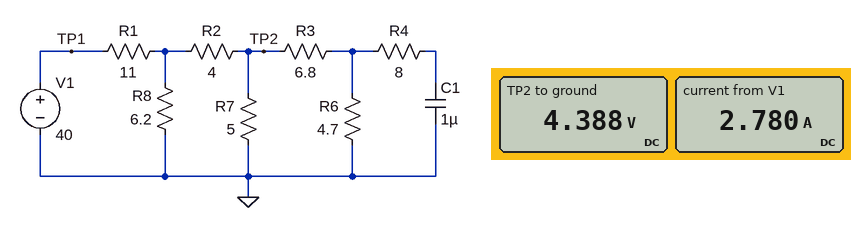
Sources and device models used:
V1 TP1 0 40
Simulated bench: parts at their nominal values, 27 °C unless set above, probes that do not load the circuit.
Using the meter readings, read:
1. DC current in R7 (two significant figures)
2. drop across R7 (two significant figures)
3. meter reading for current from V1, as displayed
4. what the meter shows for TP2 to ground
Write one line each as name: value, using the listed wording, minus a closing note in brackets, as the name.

DC current in R7: 880 mA
drop across R7: 4.4 V
meter reading for current from V1, as displayed: 2.780 A
what the meter shows for TP2 to ground: 4.388 V
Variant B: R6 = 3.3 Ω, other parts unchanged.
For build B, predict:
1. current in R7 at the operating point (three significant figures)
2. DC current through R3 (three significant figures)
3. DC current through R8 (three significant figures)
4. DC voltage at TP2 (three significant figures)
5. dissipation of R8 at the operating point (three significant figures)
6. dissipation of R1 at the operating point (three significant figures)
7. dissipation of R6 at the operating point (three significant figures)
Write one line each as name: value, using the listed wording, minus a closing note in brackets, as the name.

current in R7 at the operating point: 853 mA
DC current through R3: 422 mA
DC current through R8: 1.51 A
DC voltage at TP2: 4.26 V
dissipation of R8 at the operating point: 14.1 W
dissipation of R1 at the operating point: 85.3 W
dissipation of R6 at the operating point: 588 mW
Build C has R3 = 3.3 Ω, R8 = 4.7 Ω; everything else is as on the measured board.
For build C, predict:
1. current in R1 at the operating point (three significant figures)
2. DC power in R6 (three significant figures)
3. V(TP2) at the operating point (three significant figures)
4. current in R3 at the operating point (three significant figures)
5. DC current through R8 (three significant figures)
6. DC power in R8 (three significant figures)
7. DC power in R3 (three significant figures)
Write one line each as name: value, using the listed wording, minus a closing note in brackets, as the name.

current in R1 at the operating point: 2.89 A
DC power in R6: 927 mW
V(TP2) at the operating point: 3.55 V
current in R3 at the operating point: 444 mA
DC current through R8: 1.74 A
DC power in R8: 14.2 W
DC power in R3: 651 mW
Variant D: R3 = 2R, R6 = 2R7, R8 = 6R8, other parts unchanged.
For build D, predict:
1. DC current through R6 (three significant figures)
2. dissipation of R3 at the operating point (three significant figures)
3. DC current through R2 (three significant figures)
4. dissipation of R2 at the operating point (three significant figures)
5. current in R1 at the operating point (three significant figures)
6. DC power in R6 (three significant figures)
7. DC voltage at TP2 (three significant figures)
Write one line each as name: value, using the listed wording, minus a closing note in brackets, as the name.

DC current through R6: 741 mA
dissipation of R3 at the operating point: 1.10 W
DC current through R2: 1.44 A
dissipation of R2 at the operating point: 8.27 W
current in R1 at the operating point: 2.80 A
DC power in R6: 1.48 W
DC voltage at TP2: 3.48 V
